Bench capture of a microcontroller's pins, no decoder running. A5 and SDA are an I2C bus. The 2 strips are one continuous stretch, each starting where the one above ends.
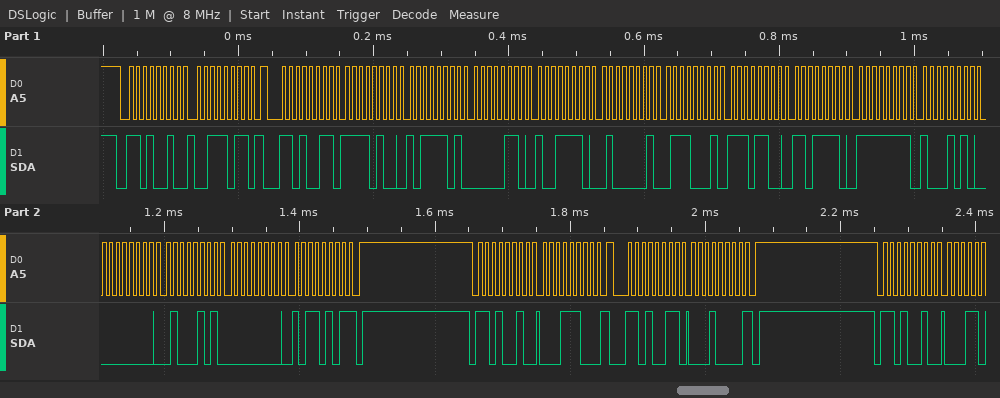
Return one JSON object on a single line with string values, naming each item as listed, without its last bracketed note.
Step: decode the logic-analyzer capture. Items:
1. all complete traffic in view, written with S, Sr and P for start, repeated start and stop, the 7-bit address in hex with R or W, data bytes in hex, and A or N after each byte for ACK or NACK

{"all complete traffic in view, written with S, Sr and P for start, repeated start and stop, the 7-bit address in hex with R or W, data bytes in hex, and A or N after each byte for ACK or NACK": "S 69W A 3B A Sr 69R A F4 A BD A 06 A 9E A 41 A 71 A EC A DE A FF A 8A A 00 A 45 A 00 A B5 N P S 69W A 1C A Sr 69R A 10 N P S 69W A"}
